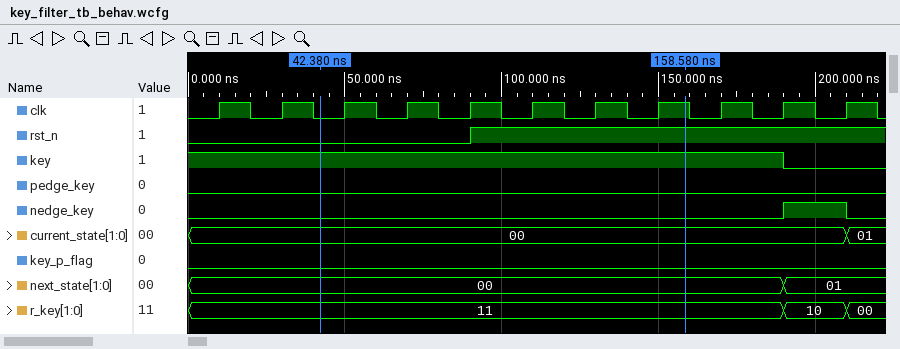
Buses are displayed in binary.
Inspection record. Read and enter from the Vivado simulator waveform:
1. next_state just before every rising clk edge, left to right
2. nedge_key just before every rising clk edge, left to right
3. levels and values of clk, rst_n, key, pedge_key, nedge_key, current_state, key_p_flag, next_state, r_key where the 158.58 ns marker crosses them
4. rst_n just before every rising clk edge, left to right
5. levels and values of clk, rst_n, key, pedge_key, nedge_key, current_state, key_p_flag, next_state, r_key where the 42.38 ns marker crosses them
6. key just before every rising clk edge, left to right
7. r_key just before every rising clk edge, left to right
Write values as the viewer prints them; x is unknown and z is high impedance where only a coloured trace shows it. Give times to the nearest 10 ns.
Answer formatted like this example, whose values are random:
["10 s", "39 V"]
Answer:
["00, 00, 00, 00, 00, 00, 00, 00, 00, 00, 01", "0 0 0 0 0 0 0 0 0 0 1", "clk=1, rst_n=1, key=1, pedge_key=0, nedge_key=0, current_state=00, key_p_flag=0, next_state=00, r_key=11", "0 0 0 0 0 1 1 1 1 1 1", "clk=0, rst_n=0, key=1, pedge_key=0, nedge_key=0, current_state=00, key_p_flag=0, next_state=00, r_key=11", "1 1 1 1 1 1 1 1 1 1 0", "11, 11, 11, 11, 11, 11, 11, 11, 11, 11, 10"]
